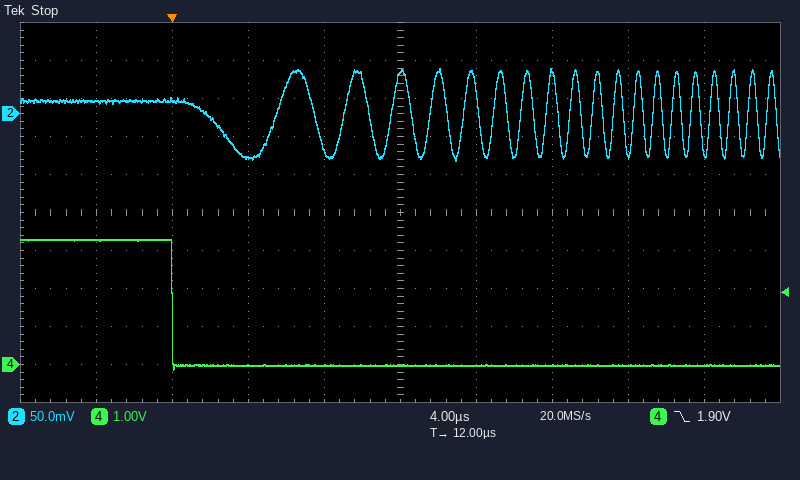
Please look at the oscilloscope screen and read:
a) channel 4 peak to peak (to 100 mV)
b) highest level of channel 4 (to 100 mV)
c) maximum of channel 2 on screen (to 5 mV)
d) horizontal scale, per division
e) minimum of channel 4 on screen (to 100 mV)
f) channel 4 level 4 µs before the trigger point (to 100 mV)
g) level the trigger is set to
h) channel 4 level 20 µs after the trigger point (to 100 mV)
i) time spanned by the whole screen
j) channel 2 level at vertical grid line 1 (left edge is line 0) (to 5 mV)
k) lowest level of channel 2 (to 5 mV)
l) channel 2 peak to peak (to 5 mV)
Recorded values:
3.4 V
3.3 V
60 mV
4 µs
-100 mV
3.3 V
1.90 V
0.0 V
40 µs
15 mV
-60 mV
120 mV
